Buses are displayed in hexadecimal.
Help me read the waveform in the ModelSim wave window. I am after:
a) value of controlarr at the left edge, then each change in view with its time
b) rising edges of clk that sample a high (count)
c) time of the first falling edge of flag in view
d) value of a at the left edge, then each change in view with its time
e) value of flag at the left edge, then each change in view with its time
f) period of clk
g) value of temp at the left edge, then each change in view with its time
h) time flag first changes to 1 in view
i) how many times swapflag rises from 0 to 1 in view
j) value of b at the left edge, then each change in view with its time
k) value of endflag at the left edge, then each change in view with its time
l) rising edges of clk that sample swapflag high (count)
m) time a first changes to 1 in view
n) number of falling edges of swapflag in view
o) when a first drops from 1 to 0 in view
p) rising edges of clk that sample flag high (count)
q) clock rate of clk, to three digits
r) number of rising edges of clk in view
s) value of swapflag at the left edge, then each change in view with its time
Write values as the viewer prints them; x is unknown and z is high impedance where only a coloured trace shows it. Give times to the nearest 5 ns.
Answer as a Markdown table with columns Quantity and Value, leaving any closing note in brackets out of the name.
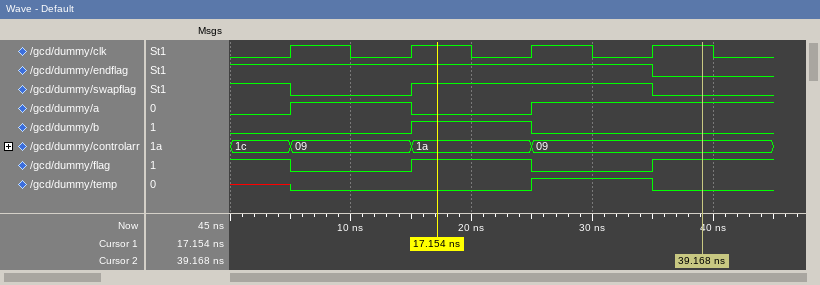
| Quantity | Value |
|---|---|
| value of controlarr at the left edge, then each change in view with its time | 1c, 09 at 5 ns, 1a at 15 ns, 09 at 25 ns |
| rising edges of clk that sample a high | 2 |
| time of the first falling edge of flag in view | 5 ns |
| value of a at the left edge, then each change in view with its time | 0, 1 at 5 ns, 0 at 15 ns, 1 at 25 ns |
| value of flag at the left edge, then each change in view with its time | 1, 0 at 5 ns, 1 at 15 ns, 0 at 25 ns, 1 at 35 ns |
| period of clk | 10 ns |
| value of temp at the left edge, then each change in view with its time | x, 0 at 5 ns, 1 at 25 ns, 0 at 35 ns |
| time flag first changes to 1 in view | 15 ns |
| how many times swapflag rises from 0 to 1 in view | 1 |
| value of b at the left edge, then each change in view with its time | 0, 1 at 15 ns, 0 at 25 ns |
| value of endflag at the left edge, then each change in view with its time | 1, 0 at 35 ns |
| rising edges of clk that sample swapflag high | 3 |
| time a first changes to 1 in view | 5 ns |
| number of falling edges of swapflag in view | 2 |
| when a first drops from 1 to 0 in view | 15 ns |
| rising edges of clk that sample flag high | 2 |
| clock rate of clk, to three digits | 100 MHz |
| number of rising edges of clk in view | 4 |
| value of swapflag at the left edge, then each change in view with its time | 1, 0 at 5 ns, 1 at 15 ns, 0 at 35 ns |
